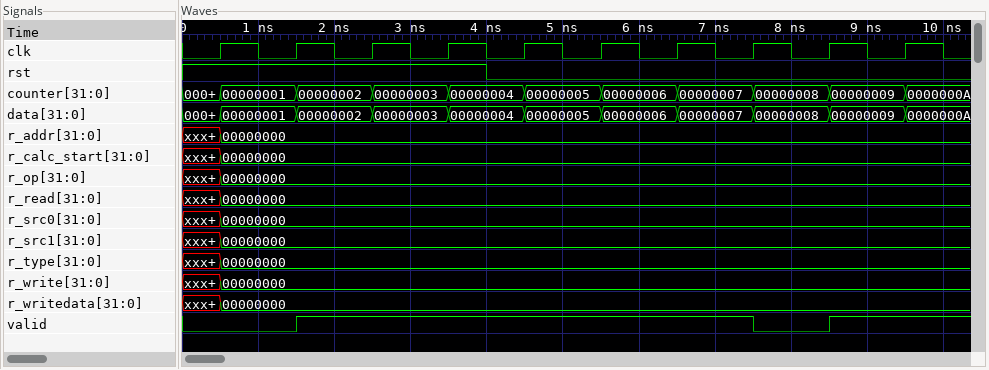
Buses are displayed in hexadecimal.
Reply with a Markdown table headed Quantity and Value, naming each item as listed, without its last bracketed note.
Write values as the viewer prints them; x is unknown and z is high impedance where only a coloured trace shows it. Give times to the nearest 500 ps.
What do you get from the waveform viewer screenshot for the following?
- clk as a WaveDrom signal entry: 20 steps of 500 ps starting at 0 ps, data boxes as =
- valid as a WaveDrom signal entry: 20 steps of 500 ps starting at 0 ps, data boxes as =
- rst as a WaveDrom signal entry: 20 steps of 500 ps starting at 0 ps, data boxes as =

| Quantity | Value |
|---|---|
| clk as a WaveDrom signal entry: 20 steps of 500 ps starting at 0 ps, data boxes as = | {name: 'clk', wave: '01010101010101010101'} |
| valid as a WaveDrom signal entry: 20 steps of 500 ps starting at 0 ps, data boxes as = | {name: 'valid', wave: '0..1...........0.1..'} |
| rst as a WaveDrom signal entry: 20 steps of 500 ps starting at 0 ps, data boxes as = | {name: 'rst', wave: '1.......0...........'} |
